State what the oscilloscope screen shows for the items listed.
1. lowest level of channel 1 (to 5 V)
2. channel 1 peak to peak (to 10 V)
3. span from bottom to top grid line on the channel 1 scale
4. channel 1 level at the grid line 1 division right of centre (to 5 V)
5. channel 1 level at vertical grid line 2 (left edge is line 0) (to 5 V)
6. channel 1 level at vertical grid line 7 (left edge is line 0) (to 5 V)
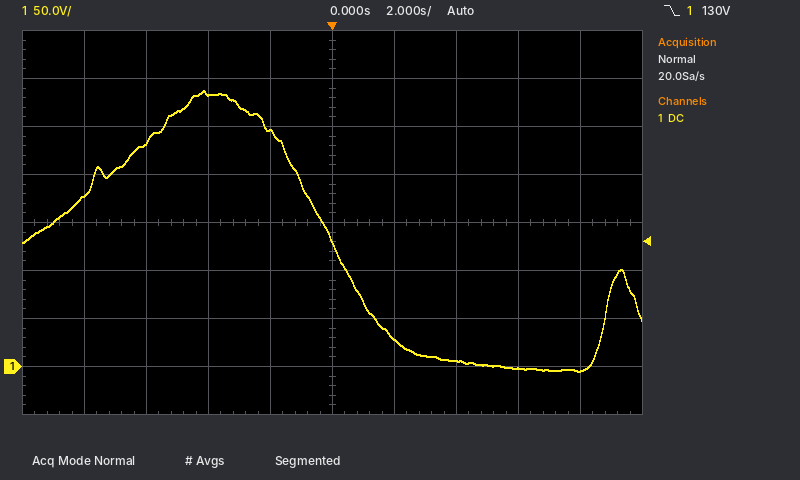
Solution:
-5 V
290 V
400 V
30 V
235 V
5 V
